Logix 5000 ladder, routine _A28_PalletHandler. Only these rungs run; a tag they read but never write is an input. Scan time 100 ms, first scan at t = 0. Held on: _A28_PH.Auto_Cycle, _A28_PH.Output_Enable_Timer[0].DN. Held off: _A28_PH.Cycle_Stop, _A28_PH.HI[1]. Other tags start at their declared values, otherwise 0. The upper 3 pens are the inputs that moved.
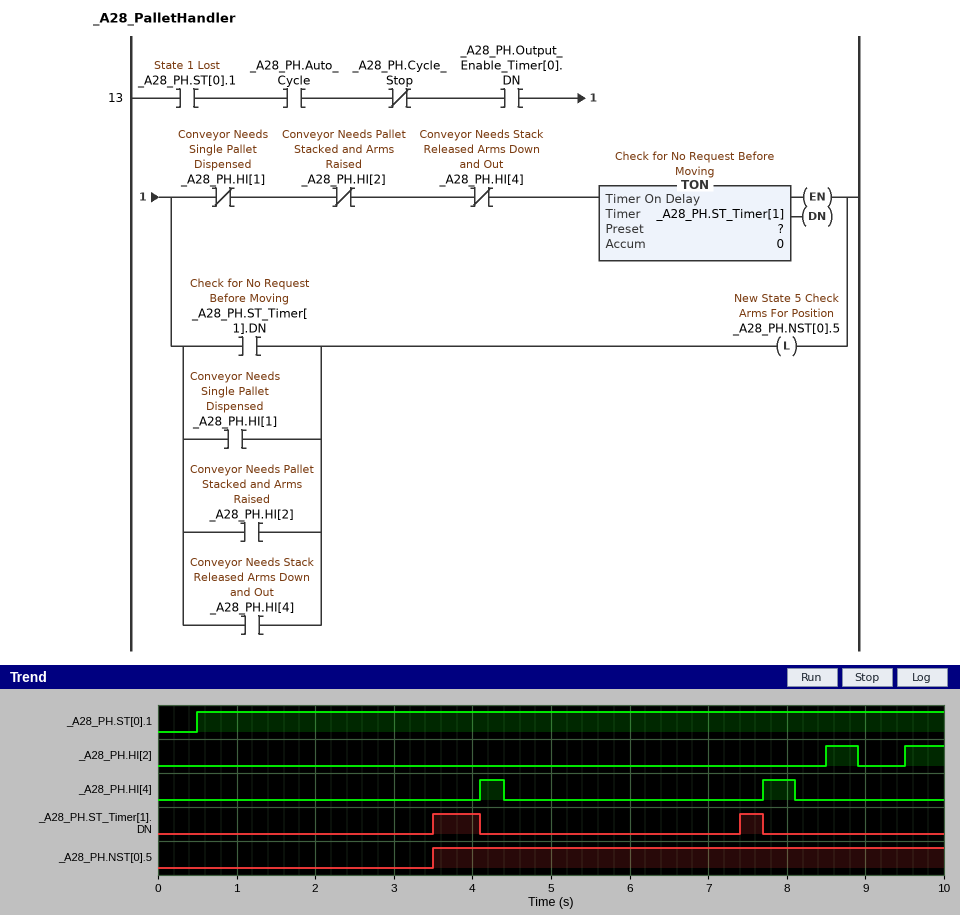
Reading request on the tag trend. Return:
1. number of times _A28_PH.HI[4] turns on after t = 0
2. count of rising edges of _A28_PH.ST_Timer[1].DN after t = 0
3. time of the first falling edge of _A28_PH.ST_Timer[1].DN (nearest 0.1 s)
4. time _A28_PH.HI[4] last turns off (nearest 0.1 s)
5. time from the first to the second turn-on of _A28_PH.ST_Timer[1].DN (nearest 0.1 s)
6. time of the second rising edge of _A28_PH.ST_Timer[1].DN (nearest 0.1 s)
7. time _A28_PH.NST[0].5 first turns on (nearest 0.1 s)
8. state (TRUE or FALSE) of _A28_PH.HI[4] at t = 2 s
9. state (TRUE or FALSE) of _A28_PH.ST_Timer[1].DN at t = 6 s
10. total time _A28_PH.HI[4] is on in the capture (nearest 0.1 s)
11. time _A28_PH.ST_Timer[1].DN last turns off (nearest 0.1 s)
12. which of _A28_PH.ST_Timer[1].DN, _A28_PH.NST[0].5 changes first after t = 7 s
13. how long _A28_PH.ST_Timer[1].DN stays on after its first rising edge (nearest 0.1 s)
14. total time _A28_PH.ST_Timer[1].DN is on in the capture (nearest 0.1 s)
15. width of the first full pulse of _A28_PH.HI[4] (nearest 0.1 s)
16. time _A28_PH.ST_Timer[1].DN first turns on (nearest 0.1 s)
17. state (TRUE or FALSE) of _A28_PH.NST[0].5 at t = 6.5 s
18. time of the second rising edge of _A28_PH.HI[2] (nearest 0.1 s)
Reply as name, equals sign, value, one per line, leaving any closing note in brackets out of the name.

number of times _A28_PH.HI[4] turns on after t = 0 = 2
count of rising edges of _A28_PH.ST_Timer[1].DN after t = 0 = 2
time of the first falling edge of _A28_PH.ST_Timer[1].DN = 4.1 s
time _A28_PH.HI[4] last turns off = 8.1 s
time from the first to the second turn-on of _A28_PH.ST_Timer[1].DN = 3.9 s
time of the second rising edge of _A28_PH.ST_Timer[1].DN = 7.4 s
time _A28_PH.NST[0].5 first turns on = 3.5 s
state (TRUE or FALSE) of _A28_PH.HI[4] at t = 2 s = FALSE
state (TRUE or FALSE) of _A28_PH.ST_Timer[1].DN at t = 6 s = FALSE
total time _A28_PH.HI[4] is on in the capture = 0.7 s
time _A28_PH.ST_Timer[1].DN last turns off = 7.7 s
which of _A28_PH.ST_Timer[1].DN, _A28_PH.NST[0].5 changes first after t = 7 s = _A28_PH.ST_Timer[1].DN
how long _A28_PH.ST_Timer[1].DN stays on after its first rising edge = 0.6 s
total time _A28_PH.ST_Timer[1].DN is on in the capture = 0.9 s
width of the first full pulse of _A28_PH.HI[4] = 0.3 s
time _A28_PH.ST_Timer[1].DN first turns on = 3.5 s
state (TRUE or FALSE) of _A28_PH.NST[0].5 at t = 6.5 s = TRUE
time of the second rising edge of _A28_PH.HI[2] = 9.5 s
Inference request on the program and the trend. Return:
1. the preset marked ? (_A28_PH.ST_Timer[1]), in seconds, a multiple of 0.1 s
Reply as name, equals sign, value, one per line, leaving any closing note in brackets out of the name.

the preset marked ? (_A28_PH.ST_Timer[1]), in seconds, a multiple of 0.1 s = 3.0 s
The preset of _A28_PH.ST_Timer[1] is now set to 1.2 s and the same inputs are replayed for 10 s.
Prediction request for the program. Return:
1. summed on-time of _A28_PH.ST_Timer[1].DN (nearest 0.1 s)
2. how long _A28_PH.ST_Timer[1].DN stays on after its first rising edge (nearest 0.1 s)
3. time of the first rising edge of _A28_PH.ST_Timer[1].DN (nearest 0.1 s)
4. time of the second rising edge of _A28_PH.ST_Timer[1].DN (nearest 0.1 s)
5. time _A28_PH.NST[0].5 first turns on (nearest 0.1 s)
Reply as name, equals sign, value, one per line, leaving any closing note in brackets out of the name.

summed on-time of _A28_PH.ST_Timer[1].DN = 4.5 s
how long _A28_PH.ST_Timer[1].DN stays on after its first rising edge = 2.4 s
time of the first rising edge of _A28_PH.ST_Timer[1].DN = 1.7 s
time of the second rising edge of _A28_PH.ST_Timer[1].DN = 5.6 s
time _A28_PH.NST[0].5 first turns on = 1.7 s
